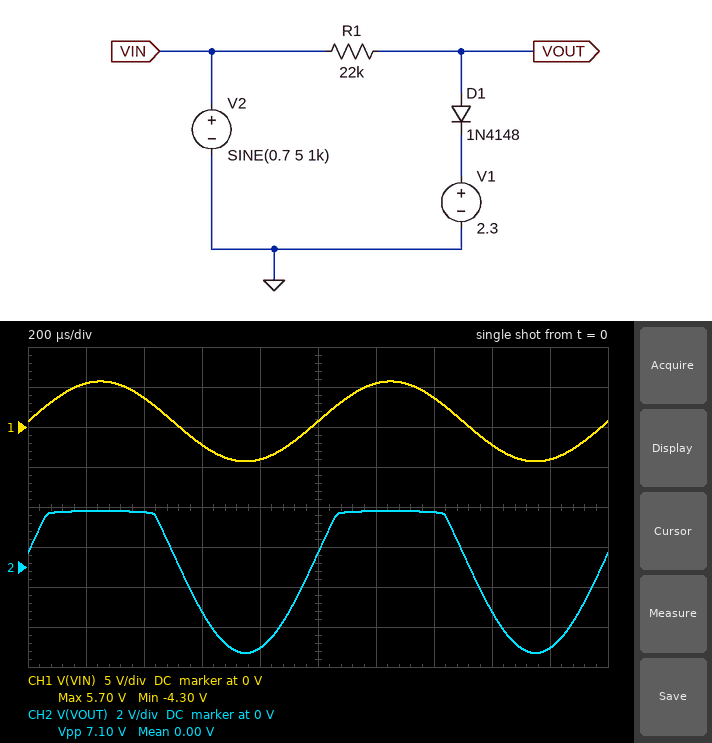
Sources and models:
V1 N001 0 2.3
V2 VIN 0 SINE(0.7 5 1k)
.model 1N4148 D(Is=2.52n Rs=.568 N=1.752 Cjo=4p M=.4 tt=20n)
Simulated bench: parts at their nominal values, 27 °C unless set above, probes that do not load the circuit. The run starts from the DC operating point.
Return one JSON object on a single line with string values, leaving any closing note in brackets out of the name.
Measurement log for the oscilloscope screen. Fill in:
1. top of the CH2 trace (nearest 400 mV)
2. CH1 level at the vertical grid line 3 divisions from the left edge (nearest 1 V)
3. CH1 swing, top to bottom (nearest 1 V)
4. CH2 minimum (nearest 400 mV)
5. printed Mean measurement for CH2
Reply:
{"top of the CH2 trace": "2.8 V", "CH1 level at the vertical grid line 3 divisions from the left edge": "-2 V", "CH1 swing, top to bottom": "10 V", "CH2 minimum": "-4.4 V", "printed Mean measurement for CH2": "0.00 V"}
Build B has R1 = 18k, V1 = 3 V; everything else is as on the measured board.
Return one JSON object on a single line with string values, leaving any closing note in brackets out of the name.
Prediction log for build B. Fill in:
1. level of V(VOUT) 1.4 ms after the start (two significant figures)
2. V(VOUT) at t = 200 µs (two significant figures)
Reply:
{"level of V(VOUT) 1.4 ms after the start": "3.4 V", "V(VOUT) at t = 200 µs": "3.5 V"}
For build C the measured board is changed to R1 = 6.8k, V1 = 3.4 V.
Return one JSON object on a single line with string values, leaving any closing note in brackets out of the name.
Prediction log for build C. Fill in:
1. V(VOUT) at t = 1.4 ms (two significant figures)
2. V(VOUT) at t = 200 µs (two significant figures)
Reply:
{"V(VOUT) at t = 1.4 ms": "3.6 V", "V(VOUT) at t = 200 µs": "3.9 V"}
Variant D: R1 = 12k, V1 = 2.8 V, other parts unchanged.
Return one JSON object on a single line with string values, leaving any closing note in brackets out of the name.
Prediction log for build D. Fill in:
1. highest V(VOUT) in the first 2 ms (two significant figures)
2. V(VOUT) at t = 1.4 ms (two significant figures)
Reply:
{"highest V(VOUT) in the first 2 ms": "3.3 V", "V(VOUT) at t = 1.4 ms": "3.2 V"}
